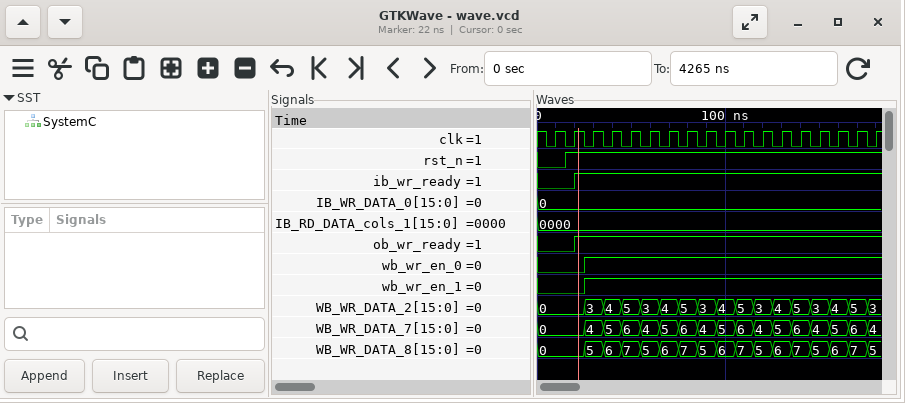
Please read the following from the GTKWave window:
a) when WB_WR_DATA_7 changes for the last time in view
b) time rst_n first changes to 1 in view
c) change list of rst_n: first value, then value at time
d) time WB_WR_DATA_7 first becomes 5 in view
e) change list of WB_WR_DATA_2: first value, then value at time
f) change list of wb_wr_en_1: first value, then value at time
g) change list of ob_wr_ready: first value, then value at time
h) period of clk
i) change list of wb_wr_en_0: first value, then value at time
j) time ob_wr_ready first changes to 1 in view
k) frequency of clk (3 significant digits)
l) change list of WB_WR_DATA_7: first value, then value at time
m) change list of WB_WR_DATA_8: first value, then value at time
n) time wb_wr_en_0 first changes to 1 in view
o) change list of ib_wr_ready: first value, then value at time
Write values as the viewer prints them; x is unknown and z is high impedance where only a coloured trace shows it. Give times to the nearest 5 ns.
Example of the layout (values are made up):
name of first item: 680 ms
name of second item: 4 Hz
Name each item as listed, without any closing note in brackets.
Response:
when WB_WR_DATA_7 changes for the last time in view: 175 ns
time rst_n first changes to 1 in view: 15 ns
change list of rst_n: first value, then value at time: 0, 1 at 15 ns
time WB_WR_DATA_7 first becomes 5 in view: 35 ns
change list of WB_WR_DATA_2: first value, then value at time: 0, 3 at 25 ns, 4 at 35 ns, 5 at 45 ns, 3 at 55 ns, 4 at 65 ns, 5 at 75 ns, 3 at 85 ns, 4 at 95 ns, 5 at 105 ns, 3 at 115 ns, 4 at 125 ns, 5 at 135 ns, 3 at 145 ns, 4 at 155 ns, 5 at 165 ns, 3 at 175 ns
change list of wb_wr_en_1: first value, then value at time: 0, 1 at 25 ns
change list of ob_wr_ready: first value, then value at time: 0, 1 at 20 ns
period of clk: 10 ns
change list of wb_wr_en_0: first value, then value at time: 0, 1 at 25 ns
time ob_wr_ready first changes to 1 in view: 20 ns
frequency of clk: 100 MHz
change list of WB_WR_DATA_7: first value, then value at time: 0, 4 at 25 ns, 5 at 35 ns, 6 at 45 ns, 4 at 55 ns, 5 at 65 ns, 6 at 75 ns, 4 at 85 ns, 5 at 95 ns, 6 at 105 ns, 4 at 115 ns, 5 at 125 ns, 6 at 135 ns, 4 at 145 ns, 5 at 155 ns, 6 at 165 ns, 4 at 175 ns
change list of WB_WR_DATA_8: first value, then value at time: 0, 5 at 25 ns, 6 at 35 ns, 7 at 45 ns, 5 at 55 ns, 6 at 65 ns, 7 at 75 ns, 5 at 85 ns, 6 at 95 ns, 7 at 105 ns, 5 at 115 ns, 6 at 125 ns, 7 at 135 ns, 5 at 145 ns, 6 at 155 ns, 7 at 165 ns, 5 at 175 ns
time wb_wr_en_0 first changes to 1 in view: 25 ns
change list of ib_wr_ready: first value, then value at time: 0, 1 at 20 ns
